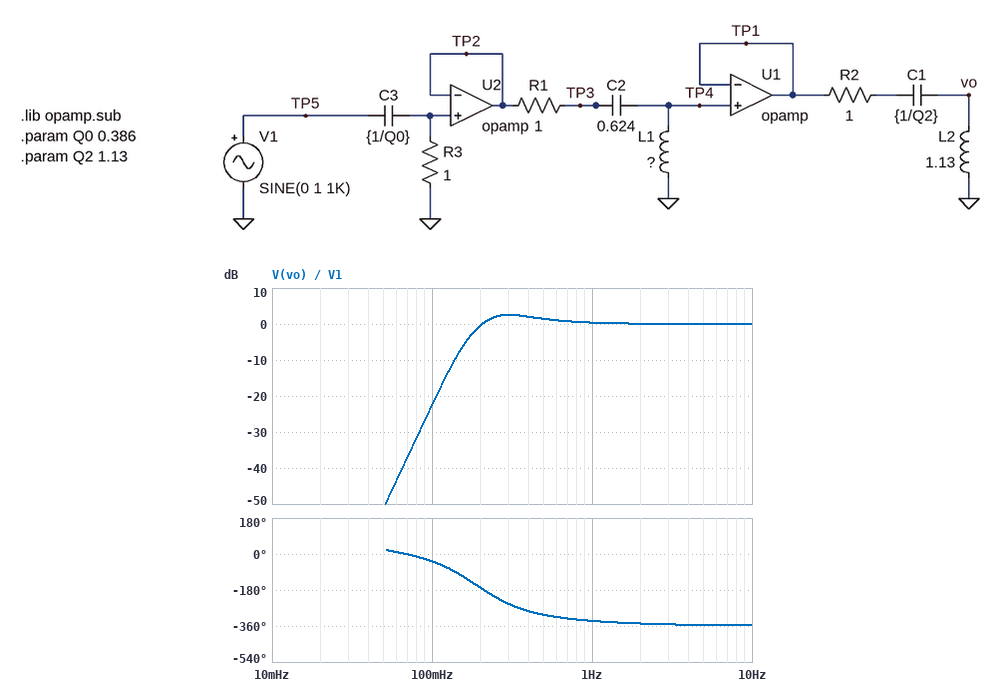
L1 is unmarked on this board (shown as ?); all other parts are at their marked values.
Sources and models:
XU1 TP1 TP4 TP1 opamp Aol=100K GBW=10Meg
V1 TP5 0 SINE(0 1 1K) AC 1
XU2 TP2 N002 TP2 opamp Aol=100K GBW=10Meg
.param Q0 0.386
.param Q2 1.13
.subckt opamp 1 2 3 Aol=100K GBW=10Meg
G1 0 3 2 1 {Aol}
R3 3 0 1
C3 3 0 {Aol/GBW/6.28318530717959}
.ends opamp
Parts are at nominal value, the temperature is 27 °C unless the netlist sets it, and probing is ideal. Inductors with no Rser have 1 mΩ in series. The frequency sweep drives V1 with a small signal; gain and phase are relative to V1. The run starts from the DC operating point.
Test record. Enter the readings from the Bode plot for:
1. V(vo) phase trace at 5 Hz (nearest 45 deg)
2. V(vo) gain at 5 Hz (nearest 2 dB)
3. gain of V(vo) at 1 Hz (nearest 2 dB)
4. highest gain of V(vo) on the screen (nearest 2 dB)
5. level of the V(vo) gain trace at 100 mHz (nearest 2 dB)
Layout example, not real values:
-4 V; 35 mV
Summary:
-360 deg; 0 dB; 0 dB; 2 dB; -22 dB
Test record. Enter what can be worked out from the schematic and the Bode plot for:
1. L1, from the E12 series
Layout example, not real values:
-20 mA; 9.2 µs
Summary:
680 mH
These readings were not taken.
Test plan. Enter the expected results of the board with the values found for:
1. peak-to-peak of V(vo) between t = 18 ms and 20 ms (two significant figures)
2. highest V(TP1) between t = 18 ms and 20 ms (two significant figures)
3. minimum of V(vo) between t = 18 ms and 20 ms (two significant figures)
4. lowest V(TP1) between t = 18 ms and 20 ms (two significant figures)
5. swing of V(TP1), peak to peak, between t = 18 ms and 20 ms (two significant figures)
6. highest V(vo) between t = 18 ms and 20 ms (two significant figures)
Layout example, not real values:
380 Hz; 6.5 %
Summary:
2.0 V; 1.0 V; -1.0 V; -1.0 V; 2.0 V; 1.0 V
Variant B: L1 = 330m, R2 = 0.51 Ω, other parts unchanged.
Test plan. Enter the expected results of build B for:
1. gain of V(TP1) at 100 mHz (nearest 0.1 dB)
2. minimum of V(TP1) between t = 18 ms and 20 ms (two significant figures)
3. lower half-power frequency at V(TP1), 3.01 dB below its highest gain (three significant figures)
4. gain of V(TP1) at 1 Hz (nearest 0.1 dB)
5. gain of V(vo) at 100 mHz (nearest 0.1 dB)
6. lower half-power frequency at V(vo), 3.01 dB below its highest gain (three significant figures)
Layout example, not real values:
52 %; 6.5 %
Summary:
-23.2 dB; -1.0 V; 347 mHz; 0 dB; -27.8 dB; 272 mHz
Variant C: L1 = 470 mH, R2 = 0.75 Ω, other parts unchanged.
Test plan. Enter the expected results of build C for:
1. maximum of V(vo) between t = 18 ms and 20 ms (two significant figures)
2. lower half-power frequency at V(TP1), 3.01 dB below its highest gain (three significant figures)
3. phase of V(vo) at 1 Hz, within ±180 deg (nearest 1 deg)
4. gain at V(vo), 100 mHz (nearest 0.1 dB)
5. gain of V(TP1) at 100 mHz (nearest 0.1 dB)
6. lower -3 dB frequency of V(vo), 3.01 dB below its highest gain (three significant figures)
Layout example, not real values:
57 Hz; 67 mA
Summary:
1.0 V; 264 mHz; 30 deg; -25.2 dB; -19.8 dB; 220 mHz
